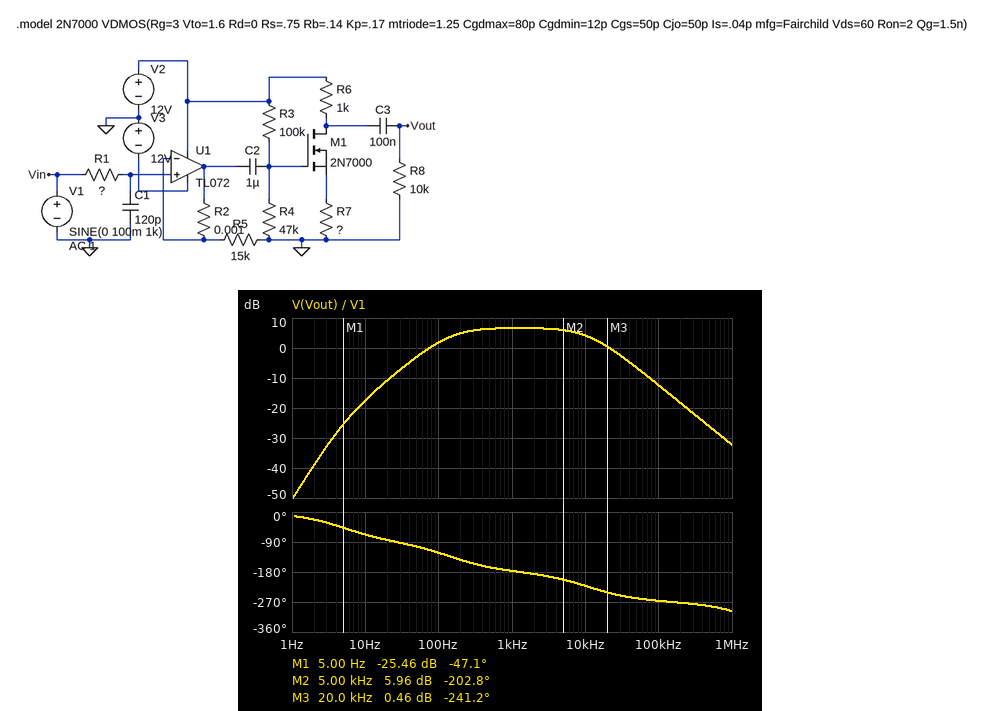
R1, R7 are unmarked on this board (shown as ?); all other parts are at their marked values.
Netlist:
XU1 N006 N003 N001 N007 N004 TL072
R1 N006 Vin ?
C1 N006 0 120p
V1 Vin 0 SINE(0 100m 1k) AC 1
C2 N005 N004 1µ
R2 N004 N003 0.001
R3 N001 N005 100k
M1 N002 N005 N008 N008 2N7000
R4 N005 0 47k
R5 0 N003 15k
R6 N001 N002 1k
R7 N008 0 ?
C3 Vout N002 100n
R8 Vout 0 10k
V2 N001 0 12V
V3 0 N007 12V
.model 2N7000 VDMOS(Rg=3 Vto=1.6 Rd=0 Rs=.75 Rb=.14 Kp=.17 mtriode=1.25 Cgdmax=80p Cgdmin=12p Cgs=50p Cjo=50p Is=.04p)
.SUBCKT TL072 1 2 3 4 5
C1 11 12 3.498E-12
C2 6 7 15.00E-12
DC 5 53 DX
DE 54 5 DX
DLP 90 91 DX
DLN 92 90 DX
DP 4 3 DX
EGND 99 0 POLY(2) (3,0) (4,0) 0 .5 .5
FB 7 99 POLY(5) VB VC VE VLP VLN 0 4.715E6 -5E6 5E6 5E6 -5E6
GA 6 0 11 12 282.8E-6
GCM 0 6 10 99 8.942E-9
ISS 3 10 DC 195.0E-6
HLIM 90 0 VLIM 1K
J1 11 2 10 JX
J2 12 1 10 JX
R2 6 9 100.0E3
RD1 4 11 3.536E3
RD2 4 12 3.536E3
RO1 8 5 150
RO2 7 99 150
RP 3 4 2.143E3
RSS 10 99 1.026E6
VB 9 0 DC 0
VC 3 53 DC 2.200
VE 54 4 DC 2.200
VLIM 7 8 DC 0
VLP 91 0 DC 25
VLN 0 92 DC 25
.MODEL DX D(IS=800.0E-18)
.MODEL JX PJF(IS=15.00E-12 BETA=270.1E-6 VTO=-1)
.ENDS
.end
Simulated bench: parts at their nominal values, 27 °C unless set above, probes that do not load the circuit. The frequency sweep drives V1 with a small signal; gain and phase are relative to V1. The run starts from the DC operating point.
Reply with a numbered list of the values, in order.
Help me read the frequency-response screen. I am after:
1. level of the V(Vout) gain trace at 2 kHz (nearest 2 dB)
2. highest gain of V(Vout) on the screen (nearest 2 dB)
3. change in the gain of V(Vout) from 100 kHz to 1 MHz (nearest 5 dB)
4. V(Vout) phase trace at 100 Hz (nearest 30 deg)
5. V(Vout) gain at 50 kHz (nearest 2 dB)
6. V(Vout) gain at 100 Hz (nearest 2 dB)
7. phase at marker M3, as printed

1. 6 dB
2. 6 dB
3. -20 dB
4. -120 deg
5. -6 dB
6. 2 dB
7. -241.2 deg
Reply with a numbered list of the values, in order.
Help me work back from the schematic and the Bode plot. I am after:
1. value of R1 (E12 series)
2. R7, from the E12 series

1. 120 kΩ
2. 390 Ω
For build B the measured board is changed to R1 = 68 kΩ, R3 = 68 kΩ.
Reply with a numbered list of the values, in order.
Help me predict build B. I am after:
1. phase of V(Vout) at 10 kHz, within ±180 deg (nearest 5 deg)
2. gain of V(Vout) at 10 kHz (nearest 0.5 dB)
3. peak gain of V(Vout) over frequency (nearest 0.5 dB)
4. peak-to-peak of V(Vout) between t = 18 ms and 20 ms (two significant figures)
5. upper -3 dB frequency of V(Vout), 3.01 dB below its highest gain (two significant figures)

1. 155 deg
2. 6.0 dB
3. 7.0 dB
4. 440 mV
5. 20 kHz
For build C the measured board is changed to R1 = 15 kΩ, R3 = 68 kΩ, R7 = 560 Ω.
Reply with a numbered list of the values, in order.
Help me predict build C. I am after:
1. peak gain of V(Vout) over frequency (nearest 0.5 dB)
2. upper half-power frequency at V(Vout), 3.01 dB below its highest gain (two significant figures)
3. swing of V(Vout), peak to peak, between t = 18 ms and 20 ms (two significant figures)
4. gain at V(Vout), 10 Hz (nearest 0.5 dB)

1. 4.0 dB
2. 89 kHz
3. 310 mV
4. -20.5 dB
